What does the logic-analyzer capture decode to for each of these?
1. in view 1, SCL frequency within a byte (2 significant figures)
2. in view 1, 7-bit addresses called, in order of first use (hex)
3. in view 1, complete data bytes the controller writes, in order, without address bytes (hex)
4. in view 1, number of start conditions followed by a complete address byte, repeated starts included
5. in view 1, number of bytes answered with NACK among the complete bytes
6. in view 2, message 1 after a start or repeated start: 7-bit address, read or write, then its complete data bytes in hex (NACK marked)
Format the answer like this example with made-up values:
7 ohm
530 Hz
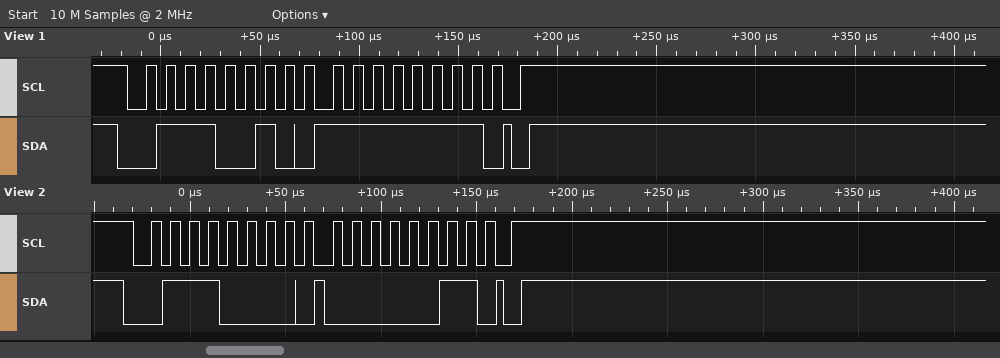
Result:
100 kHz
0x39
FF
1
0
0x38 write: 03
